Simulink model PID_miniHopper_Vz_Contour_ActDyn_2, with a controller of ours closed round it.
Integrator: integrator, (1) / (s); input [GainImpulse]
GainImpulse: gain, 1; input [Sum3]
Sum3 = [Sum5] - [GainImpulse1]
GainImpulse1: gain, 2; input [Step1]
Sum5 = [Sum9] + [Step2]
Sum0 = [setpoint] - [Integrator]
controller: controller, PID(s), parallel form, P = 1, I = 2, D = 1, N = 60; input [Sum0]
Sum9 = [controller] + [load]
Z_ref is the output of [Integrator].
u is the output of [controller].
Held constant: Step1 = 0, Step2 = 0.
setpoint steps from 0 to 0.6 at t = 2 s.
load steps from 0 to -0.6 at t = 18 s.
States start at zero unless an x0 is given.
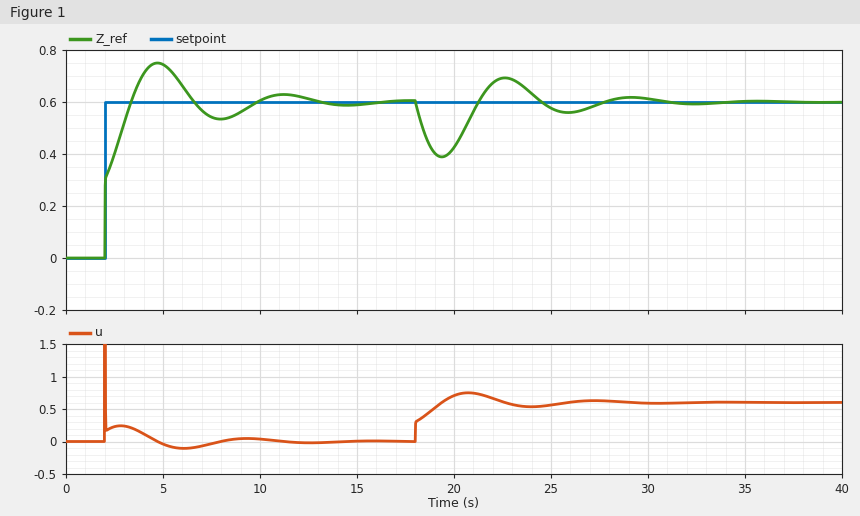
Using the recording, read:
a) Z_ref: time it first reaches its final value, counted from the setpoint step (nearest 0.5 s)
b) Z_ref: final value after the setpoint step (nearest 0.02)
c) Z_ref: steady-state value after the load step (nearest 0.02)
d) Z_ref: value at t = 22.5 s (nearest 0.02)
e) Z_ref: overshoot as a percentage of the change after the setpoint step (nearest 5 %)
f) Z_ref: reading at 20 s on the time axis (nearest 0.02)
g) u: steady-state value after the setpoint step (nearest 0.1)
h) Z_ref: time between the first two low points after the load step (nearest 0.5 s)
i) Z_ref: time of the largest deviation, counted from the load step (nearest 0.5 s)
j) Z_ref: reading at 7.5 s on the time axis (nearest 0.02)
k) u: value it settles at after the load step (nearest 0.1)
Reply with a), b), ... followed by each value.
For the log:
a) 1.5 s
b) 0.60
c) 0.60
d) 0.70
e) 25 %
f) 0.42
g) 0.0
h) 6.5 s
i) 1.5 s
j) 0.54
k) 0.6
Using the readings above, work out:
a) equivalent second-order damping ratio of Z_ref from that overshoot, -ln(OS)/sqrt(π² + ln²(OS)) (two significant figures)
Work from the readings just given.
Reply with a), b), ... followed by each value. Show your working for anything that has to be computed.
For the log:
a) ln(0.25) = -1.386; 1.386 / sqrt(9.870 + 1.922) = 0.40
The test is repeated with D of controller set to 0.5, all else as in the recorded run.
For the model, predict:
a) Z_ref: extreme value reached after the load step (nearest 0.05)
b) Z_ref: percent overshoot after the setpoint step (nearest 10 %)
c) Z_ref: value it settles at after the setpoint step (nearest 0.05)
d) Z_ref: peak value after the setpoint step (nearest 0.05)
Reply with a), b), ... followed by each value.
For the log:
a) 0.35
b) 30 %
c) 0.60
d) 0.80
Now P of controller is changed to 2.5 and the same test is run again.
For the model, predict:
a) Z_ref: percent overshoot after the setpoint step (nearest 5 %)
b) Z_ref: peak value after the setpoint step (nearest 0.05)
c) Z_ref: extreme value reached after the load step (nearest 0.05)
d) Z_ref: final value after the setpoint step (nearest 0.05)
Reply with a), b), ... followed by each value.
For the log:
a) 10 %
b) 0.65
c) 0.45
d) 0.60
